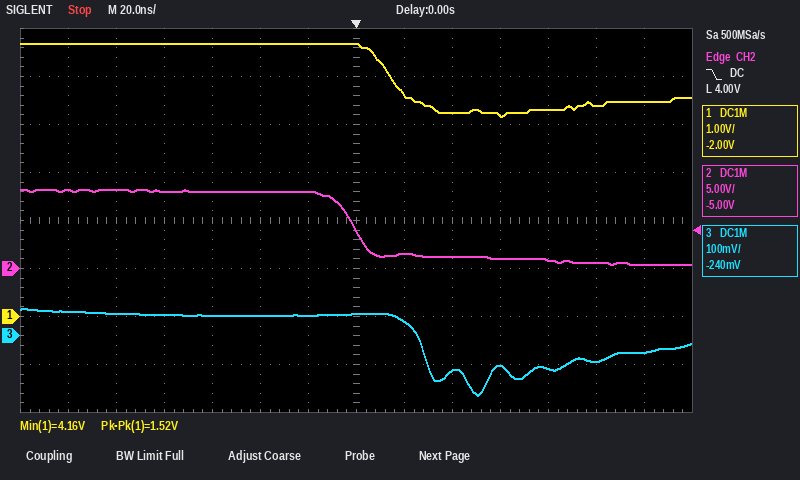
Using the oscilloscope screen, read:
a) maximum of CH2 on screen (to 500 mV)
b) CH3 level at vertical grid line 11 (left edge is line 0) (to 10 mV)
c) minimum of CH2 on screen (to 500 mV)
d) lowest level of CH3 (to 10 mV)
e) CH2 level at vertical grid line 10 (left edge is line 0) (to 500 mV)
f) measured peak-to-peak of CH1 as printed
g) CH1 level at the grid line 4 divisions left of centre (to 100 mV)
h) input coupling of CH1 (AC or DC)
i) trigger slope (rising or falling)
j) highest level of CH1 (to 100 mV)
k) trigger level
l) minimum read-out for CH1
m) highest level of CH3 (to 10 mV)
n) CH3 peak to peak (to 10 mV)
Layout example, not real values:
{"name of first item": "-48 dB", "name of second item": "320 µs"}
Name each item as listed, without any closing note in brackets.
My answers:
{"maximum of CH2 on screen": "8.0 V", "CH3 level at vertical grid line 11 (left edge is line 0)": "-70 mV", "minimum of CH2 on screen": "500 mV", "lowest level of CH3": "-120 mV", "CH2 level at vertical grid line 10 (left edge is line 0)": "1.0 V", "measured peak-to-peak of CH1 as printed": "1.52 V", "CH1 level at the grid line 4 divisions left of centre": "5.7 V", "input coupling of CH1": "DC", "trigger slope": "falling", "highest level of CH1": "5.7 V", "trigger level": "4.00 V", "minimum read-out for CH1": "4.16 V", "highest level of CH3": "60 mV", "CH3 peak to peak": "180 mV"}
